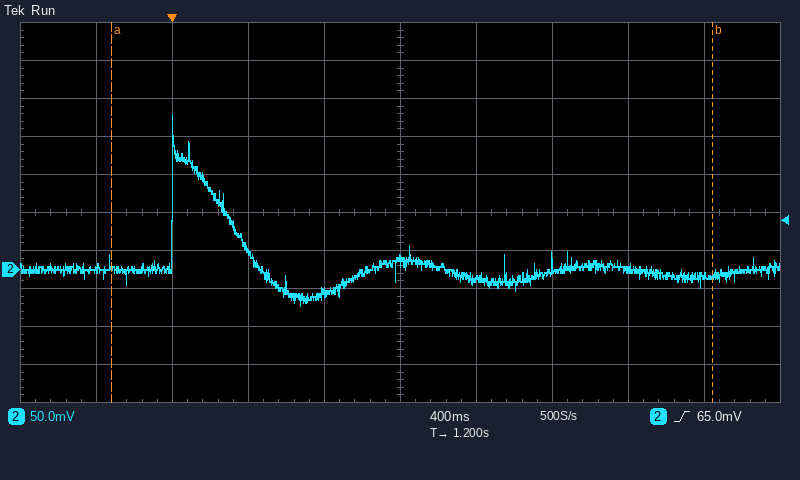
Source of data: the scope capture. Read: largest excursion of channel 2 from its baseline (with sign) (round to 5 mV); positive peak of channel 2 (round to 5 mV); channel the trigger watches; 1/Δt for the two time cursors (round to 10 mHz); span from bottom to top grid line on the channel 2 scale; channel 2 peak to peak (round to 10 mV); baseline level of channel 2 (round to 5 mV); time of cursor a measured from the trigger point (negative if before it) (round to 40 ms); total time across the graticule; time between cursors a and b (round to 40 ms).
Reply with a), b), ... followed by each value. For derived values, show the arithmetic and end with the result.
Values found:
a) 205 mV − (0 mV) = +205 mV
b) 205 mV
c) channel 2
d) 1 / 3.16 s ≈ 320 mHz
e) 500 mV
f) 250 mV
g) 0 mV
h) -320 ms
i) 4 s
j) 3.16 s
